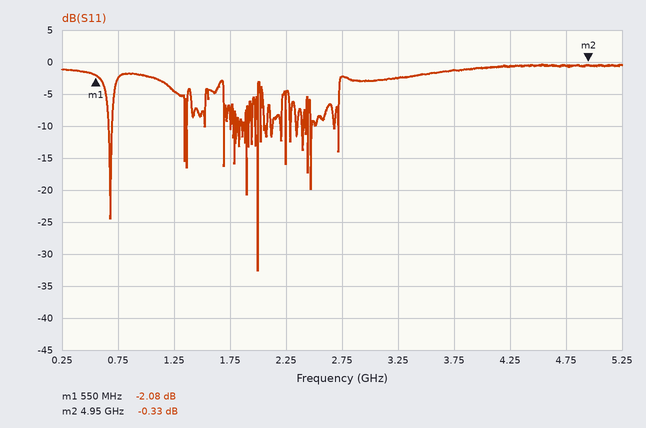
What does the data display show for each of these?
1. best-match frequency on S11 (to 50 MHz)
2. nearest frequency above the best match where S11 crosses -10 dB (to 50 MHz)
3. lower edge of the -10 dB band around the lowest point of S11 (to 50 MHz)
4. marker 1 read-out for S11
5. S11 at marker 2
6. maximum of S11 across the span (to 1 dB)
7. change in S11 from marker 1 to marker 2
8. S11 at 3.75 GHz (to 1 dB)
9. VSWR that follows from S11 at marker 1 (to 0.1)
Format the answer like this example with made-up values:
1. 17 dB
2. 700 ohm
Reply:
1. 2.00 GHz
2. 2.00 GHz
3. 2.00 GHz
4. -2.08 dB
5. -0.33 dB
6. 0 dB
7. 1.75 dB
8. -1 dB
9. 8.4
